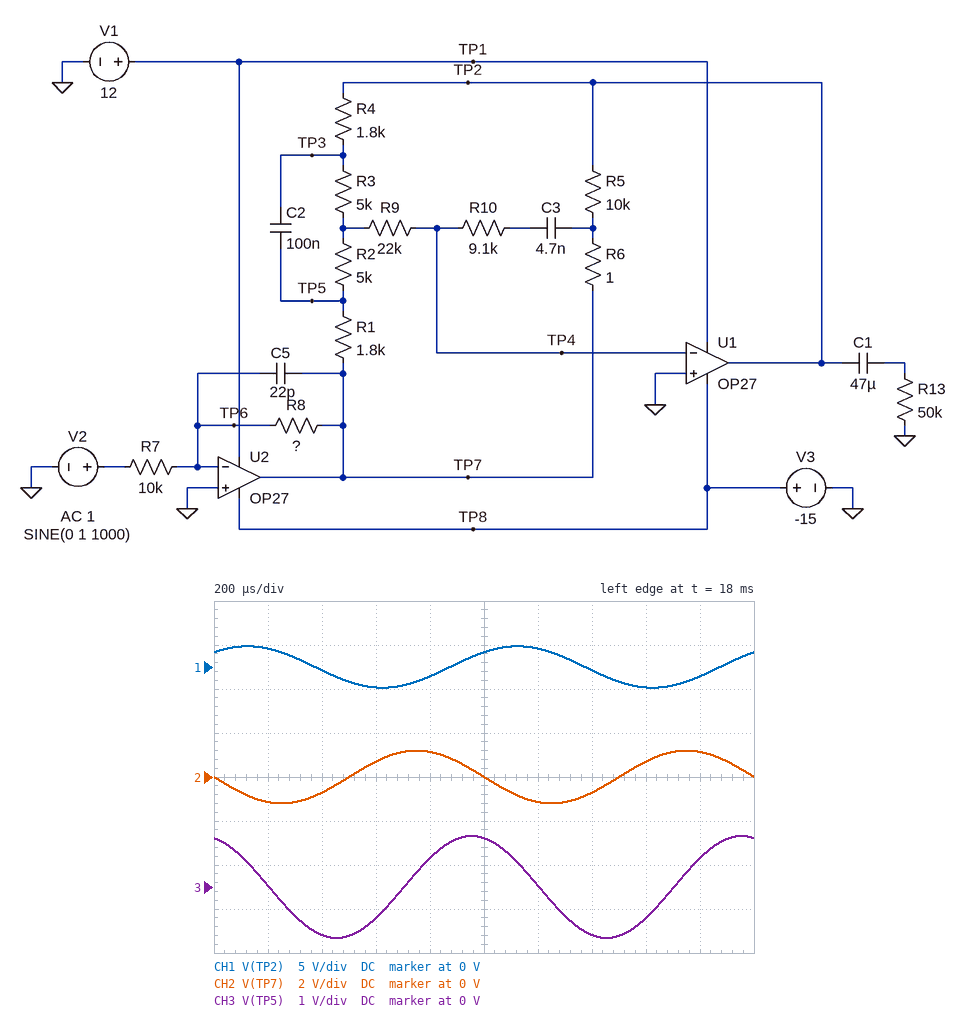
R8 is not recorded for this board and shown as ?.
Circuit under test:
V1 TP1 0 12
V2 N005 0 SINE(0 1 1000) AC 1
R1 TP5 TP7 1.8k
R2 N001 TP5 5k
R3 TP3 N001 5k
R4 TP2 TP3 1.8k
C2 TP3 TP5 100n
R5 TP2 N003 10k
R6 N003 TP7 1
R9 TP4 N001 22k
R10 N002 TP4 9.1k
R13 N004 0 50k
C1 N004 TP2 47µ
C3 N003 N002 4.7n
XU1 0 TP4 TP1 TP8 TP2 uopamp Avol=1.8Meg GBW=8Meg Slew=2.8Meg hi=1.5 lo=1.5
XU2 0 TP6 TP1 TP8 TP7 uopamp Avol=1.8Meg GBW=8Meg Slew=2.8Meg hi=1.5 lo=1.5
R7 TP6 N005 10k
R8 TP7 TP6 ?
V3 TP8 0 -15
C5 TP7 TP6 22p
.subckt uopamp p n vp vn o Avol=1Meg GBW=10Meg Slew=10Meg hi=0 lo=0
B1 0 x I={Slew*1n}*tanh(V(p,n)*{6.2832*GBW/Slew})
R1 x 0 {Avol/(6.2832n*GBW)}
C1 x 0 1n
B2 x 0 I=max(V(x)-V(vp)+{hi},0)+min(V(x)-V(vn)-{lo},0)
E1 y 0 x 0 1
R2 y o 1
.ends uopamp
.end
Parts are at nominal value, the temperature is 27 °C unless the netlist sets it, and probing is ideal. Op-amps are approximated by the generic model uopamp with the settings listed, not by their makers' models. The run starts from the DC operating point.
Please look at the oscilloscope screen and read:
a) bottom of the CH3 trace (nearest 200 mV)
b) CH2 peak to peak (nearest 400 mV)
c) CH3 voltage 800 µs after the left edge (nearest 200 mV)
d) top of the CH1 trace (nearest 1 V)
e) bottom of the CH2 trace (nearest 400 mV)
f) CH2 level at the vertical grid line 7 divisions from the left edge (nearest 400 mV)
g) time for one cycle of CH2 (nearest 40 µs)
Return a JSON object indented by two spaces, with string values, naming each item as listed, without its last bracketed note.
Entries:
{
  "bottom of the CH3 trace": "-1.2 V",
  "CH2 peak to peak": "2.4 V",
  "CH3 voltage 800 µs after the left edge": "600 mV",
  "top of the CH1 trace": "2 V",
  "bottom of the CH2 trace": "-1.2 V",
  "CH2 level at the vertical grid line 7 divisions from the left edge": "-800 mV",
  "time for one cycle of CH2": "1.00 ms"
}
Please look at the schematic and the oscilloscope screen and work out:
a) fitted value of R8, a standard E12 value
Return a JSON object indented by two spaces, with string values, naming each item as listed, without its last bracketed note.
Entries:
{
  "fitted value of R8, a standard E12 value": "12 kΩ"
}
